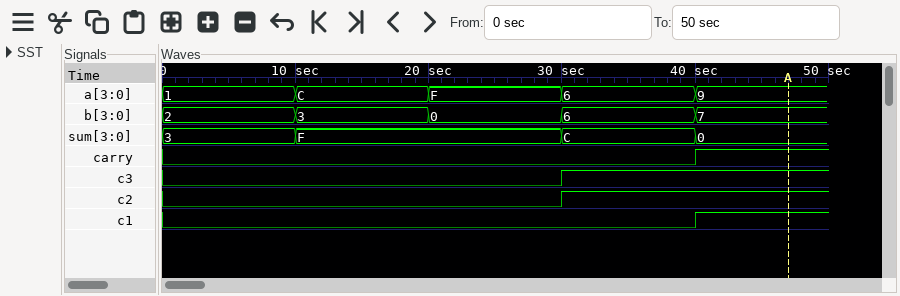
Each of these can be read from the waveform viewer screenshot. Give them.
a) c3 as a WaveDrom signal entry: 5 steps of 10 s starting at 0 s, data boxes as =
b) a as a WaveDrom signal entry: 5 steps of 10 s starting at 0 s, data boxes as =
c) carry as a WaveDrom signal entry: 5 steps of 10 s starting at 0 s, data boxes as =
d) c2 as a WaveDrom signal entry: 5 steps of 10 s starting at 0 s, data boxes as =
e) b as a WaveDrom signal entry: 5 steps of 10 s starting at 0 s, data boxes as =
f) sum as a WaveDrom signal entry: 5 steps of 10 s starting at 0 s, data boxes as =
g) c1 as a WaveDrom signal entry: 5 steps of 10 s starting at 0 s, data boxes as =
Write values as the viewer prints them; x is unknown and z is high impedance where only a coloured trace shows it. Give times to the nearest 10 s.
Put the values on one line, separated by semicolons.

{name: 'c3', wave: '0..1.'}; {name: 'a', wave: '=====', data: '1 C F 6 9'}; {name: 'carry', wave: '0...1'}; {name: 'c2', wave: '0..1.'}; {name: 'b', wave: '=====', data: '2 3 0 6 7'}; {name: 'sum', wave: '==.==', data: '3 F C 0'}; {name: 'c1', wave: '0...1'}
